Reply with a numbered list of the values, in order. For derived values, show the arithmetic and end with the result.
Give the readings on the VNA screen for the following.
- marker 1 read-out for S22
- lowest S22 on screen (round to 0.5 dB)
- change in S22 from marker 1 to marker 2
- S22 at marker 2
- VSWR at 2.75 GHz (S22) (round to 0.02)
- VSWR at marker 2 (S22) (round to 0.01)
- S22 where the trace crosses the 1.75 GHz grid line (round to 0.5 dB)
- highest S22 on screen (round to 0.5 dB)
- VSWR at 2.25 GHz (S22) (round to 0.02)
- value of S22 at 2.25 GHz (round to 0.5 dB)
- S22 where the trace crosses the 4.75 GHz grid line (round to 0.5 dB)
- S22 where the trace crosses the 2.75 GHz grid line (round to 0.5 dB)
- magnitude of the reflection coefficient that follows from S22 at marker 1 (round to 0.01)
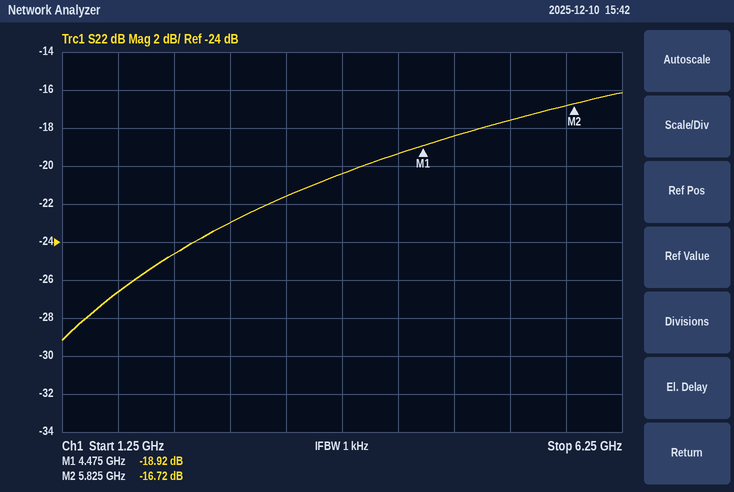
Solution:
1. -18.92 dB
2. -29.0 dB
3. -16.72 − (-18.92) = 2.20 dB
4. -16.72 dB
5. |Γ| = 10^(-23/20) = 0.0708; VSWR = (1 + 0.0708)/(1 − 0.0708) ≈ 1.15, so 1.16 to the nearest 0.02
6. (1 + 0.1459)/(1 − 0.1459) ≈ 1.34
7. -26.5 dB
8. -16.0 dB
9. |Γ| = 10^(-24.5/20) = 0.0596; VSWR = (1 + 0.0596)/(1 − 0.0596) ≈ 1.13, so 1.12 to the nearest 0.02
10. -24.5 dB
11. -18.5 dB
12. -23.0 dB
13. 10^(-18.92/20) ≈ 0.11
